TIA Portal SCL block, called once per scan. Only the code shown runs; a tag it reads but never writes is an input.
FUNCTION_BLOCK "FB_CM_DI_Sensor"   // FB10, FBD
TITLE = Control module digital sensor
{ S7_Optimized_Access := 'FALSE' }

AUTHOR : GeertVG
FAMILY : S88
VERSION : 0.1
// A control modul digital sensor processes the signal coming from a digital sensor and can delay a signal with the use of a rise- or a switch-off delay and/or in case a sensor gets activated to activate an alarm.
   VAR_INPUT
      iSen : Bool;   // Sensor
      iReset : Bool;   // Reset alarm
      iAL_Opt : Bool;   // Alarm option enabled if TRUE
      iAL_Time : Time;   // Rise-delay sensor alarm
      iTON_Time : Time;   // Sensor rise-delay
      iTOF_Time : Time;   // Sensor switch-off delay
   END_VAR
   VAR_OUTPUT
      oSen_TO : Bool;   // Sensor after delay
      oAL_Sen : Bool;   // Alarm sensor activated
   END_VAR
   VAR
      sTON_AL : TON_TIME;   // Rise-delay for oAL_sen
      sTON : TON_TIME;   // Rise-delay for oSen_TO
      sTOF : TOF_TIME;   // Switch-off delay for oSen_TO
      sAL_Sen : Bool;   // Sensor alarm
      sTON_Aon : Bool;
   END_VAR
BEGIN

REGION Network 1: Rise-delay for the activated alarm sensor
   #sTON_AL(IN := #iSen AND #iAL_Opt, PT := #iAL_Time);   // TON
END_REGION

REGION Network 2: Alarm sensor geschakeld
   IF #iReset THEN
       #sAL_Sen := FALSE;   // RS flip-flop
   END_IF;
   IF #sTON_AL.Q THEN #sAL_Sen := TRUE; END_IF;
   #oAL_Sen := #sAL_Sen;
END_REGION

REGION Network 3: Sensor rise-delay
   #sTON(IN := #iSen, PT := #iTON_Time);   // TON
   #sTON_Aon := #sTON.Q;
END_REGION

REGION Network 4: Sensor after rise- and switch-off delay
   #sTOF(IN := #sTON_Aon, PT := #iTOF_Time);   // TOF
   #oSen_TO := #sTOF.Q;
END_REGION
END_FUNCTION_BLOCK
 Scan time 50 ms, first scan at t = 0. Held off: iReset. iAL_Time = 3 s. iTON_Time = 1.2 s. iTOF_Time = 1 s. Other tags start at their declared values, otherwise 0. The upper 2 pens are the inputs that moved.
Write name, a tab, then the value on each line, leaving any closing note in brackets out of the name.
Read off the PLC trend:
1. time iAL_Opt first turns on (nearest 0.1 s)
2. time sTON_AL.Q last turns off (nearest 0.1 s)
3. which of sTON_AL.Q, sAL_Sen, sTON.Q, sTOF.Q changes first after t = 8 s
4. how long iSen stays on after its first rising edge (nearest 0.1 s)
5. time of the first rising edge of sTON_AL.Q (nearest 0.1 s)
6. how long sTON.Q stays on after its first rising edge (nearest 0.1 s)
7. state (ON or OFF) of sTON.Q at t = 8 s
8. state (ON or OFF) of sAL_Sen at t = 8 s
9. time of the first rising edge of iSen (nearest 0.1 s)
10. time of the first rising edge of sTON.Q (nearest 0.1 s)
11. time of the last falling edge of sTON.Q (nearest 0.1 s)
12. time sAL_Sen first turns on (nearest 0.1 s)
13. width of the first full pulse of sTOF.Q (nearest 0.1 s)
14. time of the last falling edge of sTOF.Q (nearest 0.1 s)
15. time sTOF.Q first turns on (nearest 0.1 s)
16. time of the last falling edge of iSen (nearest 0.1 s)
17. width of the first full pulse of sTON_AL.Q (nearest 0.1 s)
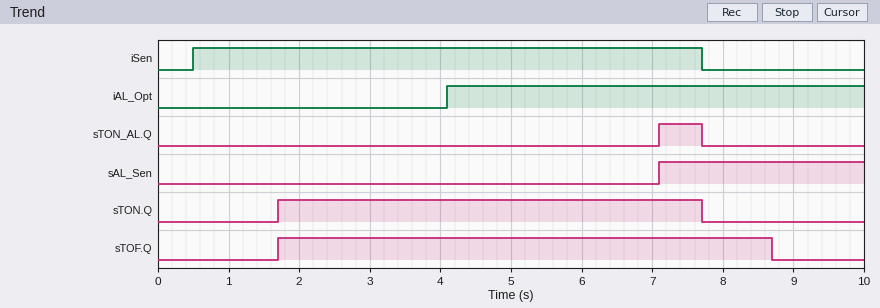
time iAL_Opt first turns on	4.1 s
time sTON_AL.Q last turns off	7.7 s
which of sTON_AL.Q, sAL_Sen, sTON.Q, sTOF.Q changes first after t = 8 s	sTOF.Q
how long iSen stays on after its first rising edge	7.2 s
time of the first rising edge of sTON_AL.Q	7.1 s
how long sTON.Q stays on after its first rising edge	6.0 s
state (ON or OFF) of sTON.Q at t = 8 s	OFF
state (ON or OFF) of sAL_Sen at t = 8 s	ON
time of the first rising edge of iSen	0.5 s
time of the first rising edge of sTON.Q	1.7 s
time of the last falling edge of sTON.Q	7.7 s
time sAL_Sen first turns on	7.1 s
width of the first full pulse of sTOF.Q	7.0 s
time of the last falling edge of sTOF.Q	8.7 s
time sTOF.Q first turns on	1.7 s
time of the last falling edge of iSen	7.7 s
width of the first full pulse of sTON_AL.Q	0.6 s
